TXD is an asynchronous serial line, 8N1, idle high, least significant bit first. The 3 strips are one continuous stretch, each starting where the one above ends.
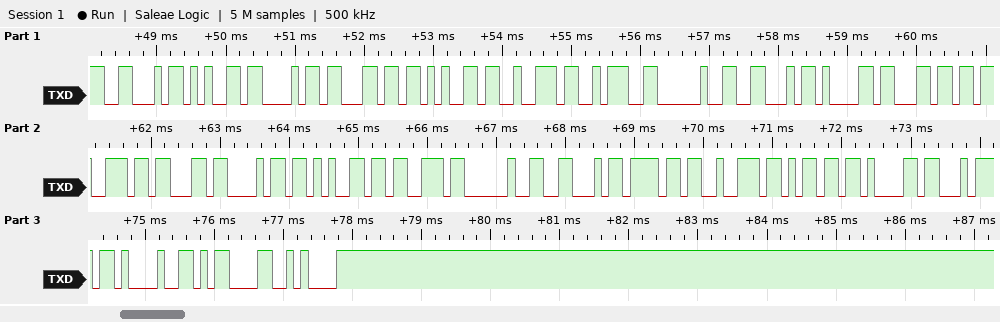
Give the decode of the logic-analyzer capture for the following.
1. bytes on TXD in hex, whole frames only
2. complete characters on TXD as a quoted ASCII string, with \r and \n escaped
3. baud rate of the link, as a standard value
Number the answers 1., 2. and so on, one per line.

1. 46 65 68 6C 65 72 3A 20 46 61 6C 73 63 68 65 73 20 46 6F 72 6D 61 74 21 0D 0A
2. "Fehler: Falsches Format!\r\n"
3. 9600 baud
